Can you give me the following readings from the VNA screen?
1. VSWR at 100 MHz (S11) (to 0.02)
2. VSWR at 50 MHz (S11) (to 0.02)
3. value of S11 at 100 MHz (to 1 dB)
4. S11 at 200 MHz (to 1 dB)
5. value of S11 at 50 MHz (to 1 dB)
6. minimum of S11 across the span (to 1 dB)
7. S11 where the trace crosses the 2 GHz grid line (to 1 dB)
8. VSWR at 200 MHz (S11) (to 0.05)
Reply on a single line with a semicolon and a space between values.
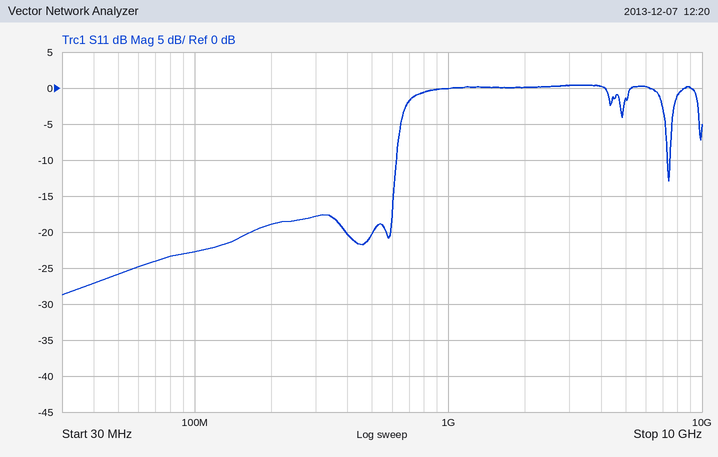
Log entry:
1.16; 1.10; -23 dB; -19 dB; -26 dB; -29 dB; 0 dB; 1.25
